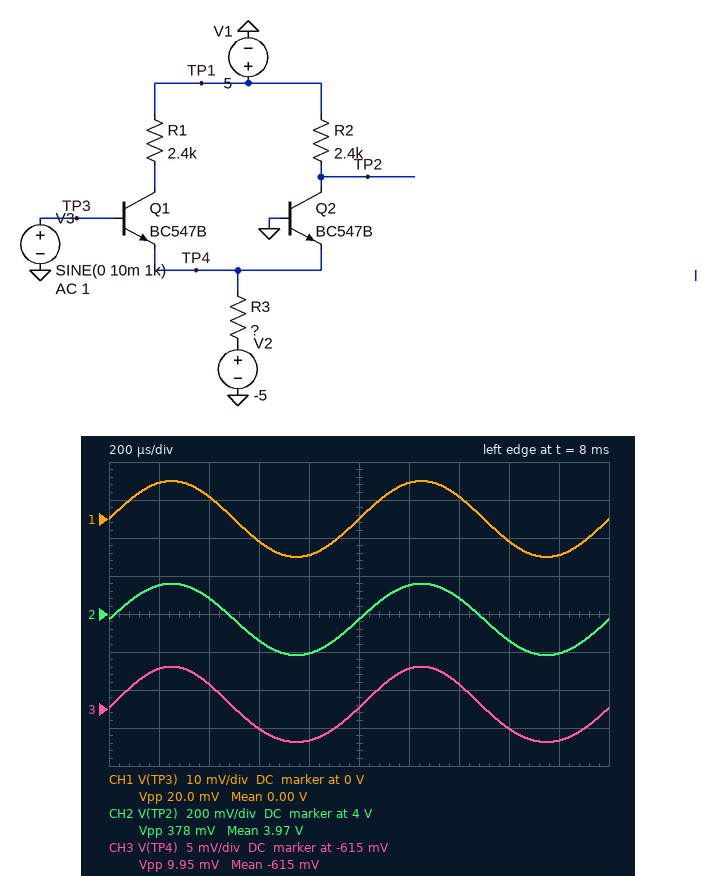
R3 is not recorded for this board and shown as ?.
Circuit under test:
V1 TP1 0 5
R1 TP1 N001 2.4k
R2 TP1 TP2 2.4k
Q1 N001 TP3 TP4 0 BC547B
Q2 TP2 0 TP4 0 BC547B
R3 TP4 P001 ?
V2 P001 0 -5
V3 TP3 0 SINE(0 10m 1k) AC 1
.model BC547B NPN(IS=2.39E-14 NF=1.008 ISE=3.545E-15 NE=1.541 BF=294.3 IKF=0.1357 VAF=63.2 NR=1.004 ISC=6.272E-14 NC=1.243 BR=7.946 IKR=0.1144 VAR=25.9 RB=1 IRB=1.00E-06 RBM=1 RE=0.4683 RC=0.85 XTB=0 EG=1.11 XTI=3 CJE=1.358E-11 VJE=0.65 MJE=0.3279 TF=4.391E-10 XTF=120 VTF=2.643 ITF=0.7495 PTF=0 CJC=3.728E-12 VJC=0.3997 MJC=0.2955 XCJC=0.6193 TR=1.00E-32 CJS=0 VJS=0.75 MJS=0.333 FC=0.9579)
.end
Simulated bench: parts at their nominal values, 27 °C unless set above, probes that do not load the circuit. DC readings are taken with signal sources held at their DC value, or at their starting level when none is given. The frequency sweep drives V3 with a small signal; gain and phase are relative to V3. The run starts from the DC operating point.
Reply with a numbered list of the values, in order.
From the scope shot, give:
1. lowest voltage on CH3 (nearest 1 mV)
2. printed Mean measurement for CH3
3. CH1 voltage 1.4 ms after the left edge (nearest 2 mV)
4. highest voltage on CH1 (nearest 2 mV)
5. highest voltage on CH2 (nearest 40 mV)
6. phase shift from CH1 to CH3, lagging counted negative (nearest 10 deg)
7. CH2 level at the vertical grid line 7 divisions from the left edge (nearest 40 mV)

1. -619 mV
2. -615 mV
3. 6 mV
4. 10 mV
5. 4.16 V
6. 0 deg
7. 4.08 V
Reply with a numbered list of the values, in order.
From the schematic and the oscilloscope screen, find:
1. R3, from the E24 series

1. 5.1 kΩ
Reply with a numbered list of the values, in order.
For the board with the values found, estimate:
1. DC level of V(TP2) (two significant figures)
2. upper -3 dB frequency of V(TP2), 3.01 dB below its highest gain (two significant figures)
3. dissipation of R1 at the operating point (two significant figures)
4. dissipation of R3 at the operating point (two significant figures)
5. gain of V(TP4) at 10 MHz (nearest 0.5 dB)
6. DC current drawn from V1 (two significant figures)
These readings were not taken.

1. 4.0 V
2. 36 MHz
3. 440 µW
4. 3.8 mW
5. -6.0 dB
6. 860 µA
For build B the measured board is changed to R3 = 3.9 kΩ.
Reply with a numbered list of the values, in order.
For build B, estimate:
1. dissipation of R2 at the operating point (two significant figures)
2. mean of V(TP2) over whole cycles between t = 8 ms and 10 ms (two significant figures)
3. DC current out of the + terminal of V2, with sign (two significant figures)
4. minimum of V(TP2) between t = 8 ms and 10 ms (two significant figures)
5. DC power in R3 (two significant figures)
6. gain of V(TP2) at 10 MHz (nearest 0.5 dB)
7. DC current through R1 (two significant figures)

1. 750 µW
2. 3.7 V
3. -1.1 mA
4. 3.4 V
5. 4.9 mW
6. 27.5 dB
7. 560 µA
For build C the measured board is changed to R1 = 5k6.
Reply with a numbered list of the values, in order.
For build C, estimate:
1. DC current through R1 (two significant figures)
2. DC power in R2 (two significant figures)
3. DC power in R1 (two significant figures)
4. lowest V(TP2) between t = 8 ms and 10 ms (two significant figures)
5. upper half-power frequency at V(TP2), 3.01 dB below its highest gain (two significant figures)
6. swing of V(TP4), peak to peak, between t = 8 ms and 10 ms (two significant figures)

1. 420 µA
2. 450 µW
3. 1.0 mW
4. 3.8 V
5. 37 MHz
6. 9.7 mV
